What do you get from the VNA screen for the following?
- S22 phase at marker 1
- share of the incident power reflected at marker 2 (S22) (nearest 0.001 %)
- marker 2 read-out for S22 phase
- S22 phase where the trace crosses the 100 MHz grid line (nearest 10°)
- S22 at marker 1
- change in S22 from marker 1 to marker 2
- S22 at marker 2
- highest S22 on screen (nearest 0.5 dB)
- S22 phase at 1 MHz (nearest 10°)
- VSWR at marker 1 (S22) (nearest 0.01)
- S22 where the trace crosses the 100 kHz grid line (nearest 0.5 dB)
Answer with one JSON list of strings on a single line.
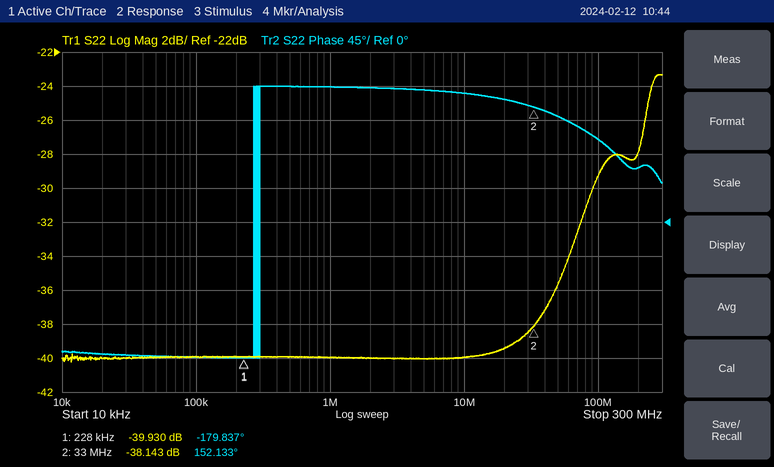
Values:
["-179.837°", "0.015 %", "152.133°", "110°", "-39.930 dB", "1.787 dB", "-38.143 dB", "-23.5 dB", "180°", "1.02", "-40.0 dB"]
